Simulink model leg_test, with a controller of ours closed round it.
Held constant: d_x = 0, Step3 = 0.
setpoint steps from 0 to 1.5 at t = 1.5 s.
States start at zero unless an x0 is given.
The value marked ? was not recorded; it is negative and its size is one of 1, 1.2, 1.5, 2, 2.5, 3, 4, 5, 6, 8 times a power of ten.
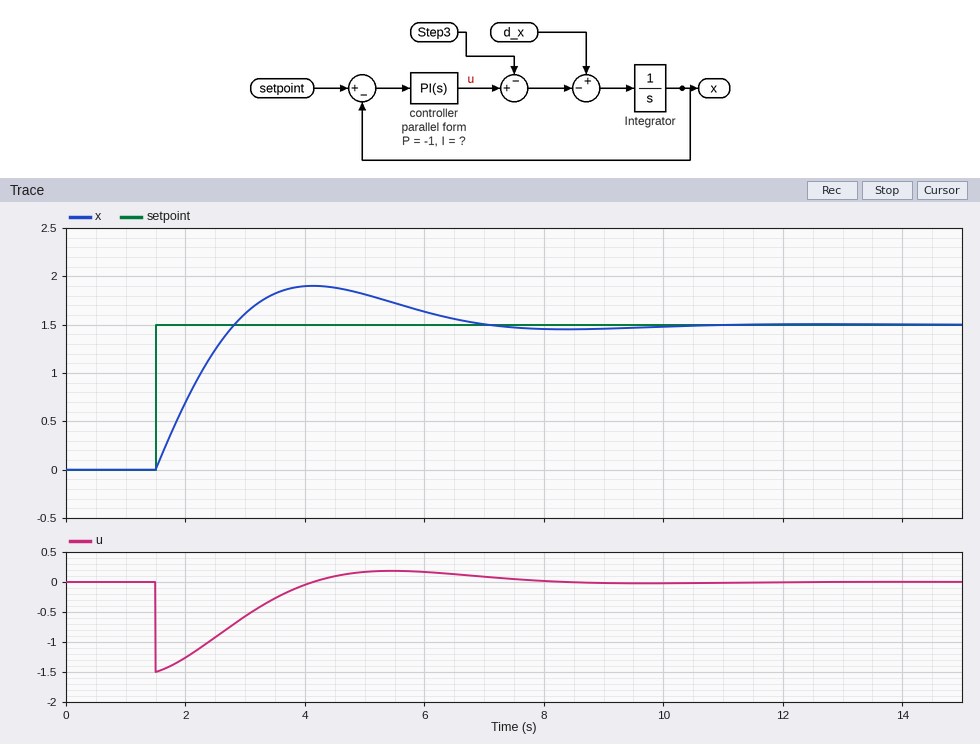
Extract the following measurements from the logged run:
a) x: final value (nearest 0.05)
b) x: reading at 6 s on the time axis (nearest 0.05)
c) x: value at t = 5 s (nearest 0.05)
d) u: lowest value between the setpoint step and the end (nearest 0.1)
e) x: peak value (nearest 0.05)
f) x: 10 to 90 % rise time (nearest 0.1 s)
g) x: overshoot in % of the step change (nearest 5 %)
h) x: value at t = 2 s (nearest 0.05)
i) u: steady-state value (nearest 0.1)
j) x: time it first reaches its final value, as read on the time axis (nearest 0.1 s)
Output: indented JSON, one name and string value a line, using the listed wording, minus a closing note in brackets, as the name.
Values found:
{
  "x: final value": "1.50",
  "x: reading at 6 s on the time axis": "1.65",
  "x: value at t = 5 s": "1.80",
  "u: lowest value between the setpoint step and the end": "-1.5",
  "x: peak value": "1.90",
  "x: 10 to 90 % rise time": "1.0 s",
  "x: overshoot in % of the step change": "25 %",
  "x: value at t = 2 s": "0.70",
  "u: steady-state value": "0.0",
  "x: time it first reaches its final value, as read on the time axis": "2.8 s"
}
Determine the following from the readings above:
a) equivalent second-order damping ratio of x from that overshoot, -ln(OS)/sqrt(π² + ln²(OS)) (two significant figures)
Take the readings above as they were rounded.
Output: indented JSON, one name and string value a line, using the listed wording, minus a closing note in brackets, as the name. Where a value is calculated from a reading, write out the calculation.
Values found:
{
  "equivalent second-order damping ratio of x from that overshoot, -ln(OS)/sqrt(π² + ln²(OS))": "ln(0.25) = -1.386; 1.386 / sqrt(9.870 + 1.922) = 0.40"
}
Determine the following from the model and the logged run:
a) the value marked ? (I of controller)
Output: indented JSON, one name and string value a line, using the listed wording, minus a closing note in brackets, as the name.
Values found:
{
  "the value marked ?": "-0.8"
}
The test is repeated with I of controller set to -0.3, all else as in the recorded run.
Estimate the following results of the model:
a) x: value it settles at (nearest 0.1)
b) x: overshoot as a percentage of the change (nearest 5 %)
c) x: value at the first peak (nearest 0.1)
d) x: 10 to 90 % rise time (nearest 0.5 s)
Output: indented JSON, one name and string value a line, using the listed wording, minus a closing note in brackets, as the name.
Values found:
{
  "x: value it settles at": "1.5",
  "x: overshoot as a percentage of the change": "15 %",
  "x: value at the first peak": "1.7",
  "x: 10 to 90 % rise time": "1.5 s"
}
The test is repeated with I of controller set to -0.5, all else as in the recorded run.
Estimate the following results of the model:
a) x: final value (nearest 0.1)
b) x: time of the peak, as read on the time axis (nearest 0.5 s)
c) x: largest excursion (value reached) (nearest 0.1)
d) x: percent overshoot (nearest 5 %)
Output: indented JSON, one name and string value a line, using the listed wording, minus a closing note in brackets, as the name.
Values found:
{
  "x: final value": "1.5",
  "x: time of the peak, as read on the time axis": "4.5 s",
  "x: largest excursion (value reached)": "1.8",
  "x: percent overshoot": "20 %"
}
